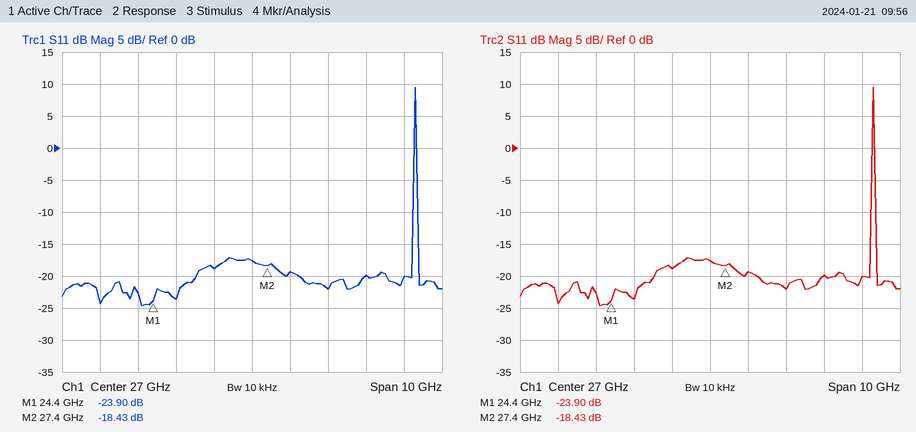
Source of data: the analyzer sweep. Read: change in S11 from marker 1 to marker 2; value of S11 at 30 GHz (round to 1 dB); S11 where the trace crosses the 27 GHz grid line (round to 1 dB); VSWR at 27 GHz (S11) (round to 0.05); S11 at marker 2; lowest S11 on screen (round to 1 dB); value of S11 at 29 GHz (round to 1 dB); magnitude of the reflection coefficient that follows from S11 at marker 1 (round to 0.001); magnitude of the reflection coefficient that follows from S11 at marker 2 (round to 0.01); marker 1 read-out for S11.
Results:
5.47 dB
-20 dB
-18 dB
1.30
-18.43 dB
-25 dB
-22 dB
0.064
0.12
-23.90 dB
